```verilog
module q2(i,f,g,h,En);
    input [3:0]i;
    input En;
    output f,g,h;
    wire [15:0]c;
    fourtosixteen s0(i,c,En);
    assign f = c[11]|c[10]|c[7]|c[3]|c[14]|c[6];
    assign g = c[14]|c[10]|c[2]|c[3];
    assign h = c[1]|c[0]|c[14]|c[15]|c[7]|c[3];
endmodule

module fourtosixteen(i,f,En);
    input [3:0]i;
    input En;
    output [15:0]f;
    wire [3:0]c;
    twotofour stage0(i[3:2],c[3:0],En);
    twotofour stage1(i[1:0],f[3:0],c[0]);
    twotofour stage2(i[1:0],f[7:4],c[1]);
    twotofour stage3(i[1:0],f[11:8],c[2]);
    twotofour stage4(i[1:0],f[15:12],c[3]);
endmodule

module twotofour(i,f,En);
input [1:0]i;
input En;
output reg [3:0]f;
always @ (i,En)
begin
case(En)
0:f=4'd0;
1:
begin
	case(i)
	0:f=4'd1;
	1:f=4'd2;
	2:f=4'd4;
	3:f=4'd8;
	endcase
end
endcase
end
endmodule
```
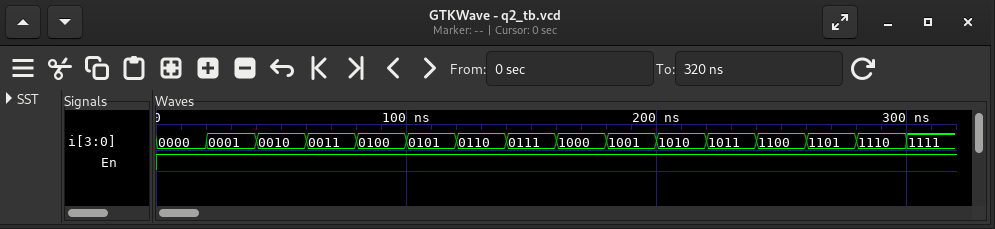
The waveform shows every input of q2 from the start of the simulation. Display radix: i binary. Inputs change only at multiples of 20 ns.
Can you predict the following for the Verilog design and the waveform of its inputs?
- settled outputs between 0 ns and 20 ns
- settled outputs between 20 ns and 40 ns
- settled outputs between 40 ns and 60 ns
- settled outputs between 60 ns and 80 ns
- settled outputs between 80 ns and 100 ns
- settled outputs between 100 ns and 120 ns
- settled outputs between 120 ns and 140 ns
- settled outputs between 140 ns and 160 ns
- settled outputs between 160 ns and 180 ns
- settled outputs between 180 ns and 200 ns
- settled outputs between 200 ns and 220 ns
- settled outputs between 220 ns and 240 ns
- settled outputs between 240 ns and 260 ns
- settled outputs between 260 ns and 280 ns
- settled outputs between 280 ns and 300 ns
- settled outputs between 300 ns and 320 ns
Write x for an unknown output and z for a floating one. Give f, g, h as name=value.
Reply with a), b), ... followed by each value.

a) f=0, g=0, h=1
b) f=0, g=0, h=1
c) f=0, g=1, h=0
d) f=1, g=1, h=1
e) f=0, g=0, h=0
f) f=0, g=0, h=0
g) f=1, g=0, h=0
h) f=1, g=0, h=1
i) f=0, g=0, h=0
j) f=0, g=0, h=0
k) f=1, g=1, h=0
l) f=1, g=0, h=0
m) f=0, g=0, h=0
n) f=0, g=0, h=0
o) f=1, g=1, h=1
p) f=0, g=0, h=1
